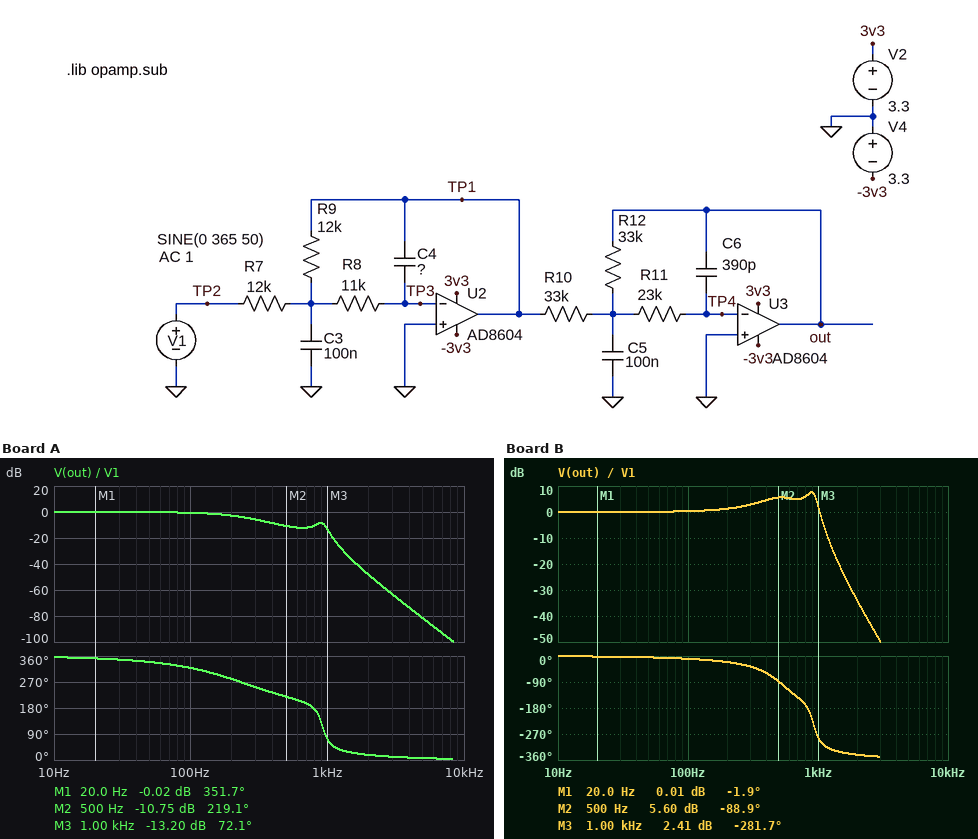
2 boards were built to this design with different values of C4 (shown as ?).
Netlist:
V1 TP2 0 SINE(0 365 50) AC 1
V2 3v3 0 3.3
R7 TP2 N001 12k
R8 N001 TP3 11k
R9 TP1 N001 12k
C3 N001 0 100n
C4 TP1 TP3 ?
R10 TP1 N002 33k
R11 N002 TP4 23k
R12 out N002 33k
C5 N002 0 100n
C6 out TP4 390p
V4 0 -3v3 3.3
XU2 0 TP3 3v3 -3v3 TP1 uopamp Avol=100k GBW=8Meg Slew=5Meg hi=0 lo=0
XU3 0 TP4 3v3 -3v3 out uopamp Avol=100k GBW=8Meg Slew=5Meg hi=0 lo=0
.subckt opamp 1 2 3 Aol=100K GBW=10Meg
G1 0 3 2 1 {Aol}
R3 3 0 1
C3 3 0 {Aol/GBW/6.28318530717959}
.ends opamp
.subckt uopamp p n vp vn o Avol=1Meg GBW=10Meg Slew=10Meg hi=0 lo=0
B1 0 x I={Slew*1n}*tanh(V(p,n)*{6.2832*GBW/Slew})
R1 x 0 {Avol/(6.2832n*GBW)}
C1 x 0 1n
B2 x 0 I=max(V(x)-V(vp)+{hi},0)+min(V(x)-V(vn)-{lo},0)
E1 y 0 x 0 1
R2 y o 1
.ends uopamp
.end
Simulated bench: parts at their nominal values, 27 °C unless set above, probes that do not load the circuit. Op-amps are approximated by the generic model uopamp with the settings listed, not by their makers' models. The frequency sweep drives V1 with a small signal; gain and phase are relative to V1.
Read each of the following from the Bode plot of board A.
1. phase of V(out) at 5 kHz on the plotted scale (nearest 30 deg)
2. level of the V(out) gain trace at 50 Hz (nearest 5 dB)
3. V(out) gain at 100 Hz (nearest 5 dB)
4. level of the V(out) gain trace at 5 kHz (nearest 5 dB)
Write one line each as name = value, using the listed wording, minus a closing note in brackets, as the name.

phase of V(out) at 5 kHz on the plotted scale = 0 deg
level of the V(out) gain trace at 50 Hz = 0 dB
V(out) gain at 100 Hz = 0 dB
level of the V(out) gain trace at 5 kHz = -80 dB
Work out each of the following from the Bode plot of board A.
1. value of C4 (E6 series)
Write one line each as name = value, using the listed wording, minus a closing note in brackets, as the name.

value of C4 = 33 nF
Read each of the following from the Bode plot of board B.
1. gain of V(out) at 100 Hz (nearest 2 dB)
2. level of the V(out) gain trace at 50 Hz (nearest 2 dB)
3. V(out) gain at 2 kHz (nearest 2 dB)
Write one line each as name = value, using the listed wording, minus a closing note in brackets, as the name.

gain of V(out) at 100 Hz = 0 dB
level of the V(out) gain trace at 50 Hz = 0 dB
V(out) gain at 2 kHz = -34 dB
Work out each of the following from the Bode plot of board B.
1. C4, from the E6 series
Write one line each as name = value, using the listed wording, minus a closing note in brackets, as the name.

C4, from the E6 series = 6.8 nF
